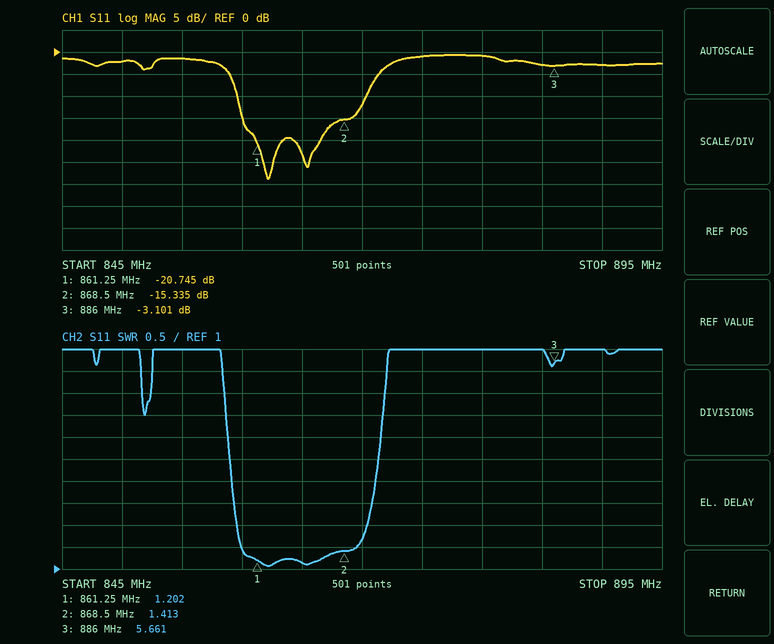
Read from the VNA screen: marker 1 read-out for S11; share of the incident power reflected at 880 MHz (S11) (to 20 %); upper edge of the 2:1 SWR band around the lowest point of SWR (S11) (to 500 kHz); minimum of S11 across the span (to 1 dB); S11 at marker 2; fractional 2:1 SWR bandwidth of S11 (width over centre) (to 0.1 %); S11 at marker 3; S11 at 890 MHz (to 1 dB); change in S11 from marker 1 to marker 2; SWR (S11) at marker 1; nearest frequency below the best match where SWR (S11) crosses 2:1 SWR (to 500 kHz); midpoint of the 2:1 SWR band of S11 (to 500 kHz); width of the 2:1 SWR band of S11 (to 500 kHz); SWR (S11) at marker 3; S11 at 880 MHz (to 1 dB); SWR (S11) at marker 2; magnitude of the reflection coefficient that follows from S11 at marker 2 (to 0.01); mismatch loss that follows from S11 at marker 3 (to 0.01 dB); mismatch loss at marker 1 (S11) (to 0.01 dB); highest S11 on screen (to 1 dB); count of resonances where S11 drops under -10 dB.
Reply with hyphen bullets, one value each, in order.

- -20.745 dB
- 80 %
- 870.5 MHz
- -29 dB
- -15.335 dB
- 1.3 %
- -3.101 dB
- -3 dB
- 5.410 dB
- 1.202
- 859.5 MHz
- 865.0 MHz
- 11.0 MHz
- 5.661
- -1 dB
- 1.413
- 0.17
- 2.92 dB
- 0.04 dB
- -1 dB
- 2
